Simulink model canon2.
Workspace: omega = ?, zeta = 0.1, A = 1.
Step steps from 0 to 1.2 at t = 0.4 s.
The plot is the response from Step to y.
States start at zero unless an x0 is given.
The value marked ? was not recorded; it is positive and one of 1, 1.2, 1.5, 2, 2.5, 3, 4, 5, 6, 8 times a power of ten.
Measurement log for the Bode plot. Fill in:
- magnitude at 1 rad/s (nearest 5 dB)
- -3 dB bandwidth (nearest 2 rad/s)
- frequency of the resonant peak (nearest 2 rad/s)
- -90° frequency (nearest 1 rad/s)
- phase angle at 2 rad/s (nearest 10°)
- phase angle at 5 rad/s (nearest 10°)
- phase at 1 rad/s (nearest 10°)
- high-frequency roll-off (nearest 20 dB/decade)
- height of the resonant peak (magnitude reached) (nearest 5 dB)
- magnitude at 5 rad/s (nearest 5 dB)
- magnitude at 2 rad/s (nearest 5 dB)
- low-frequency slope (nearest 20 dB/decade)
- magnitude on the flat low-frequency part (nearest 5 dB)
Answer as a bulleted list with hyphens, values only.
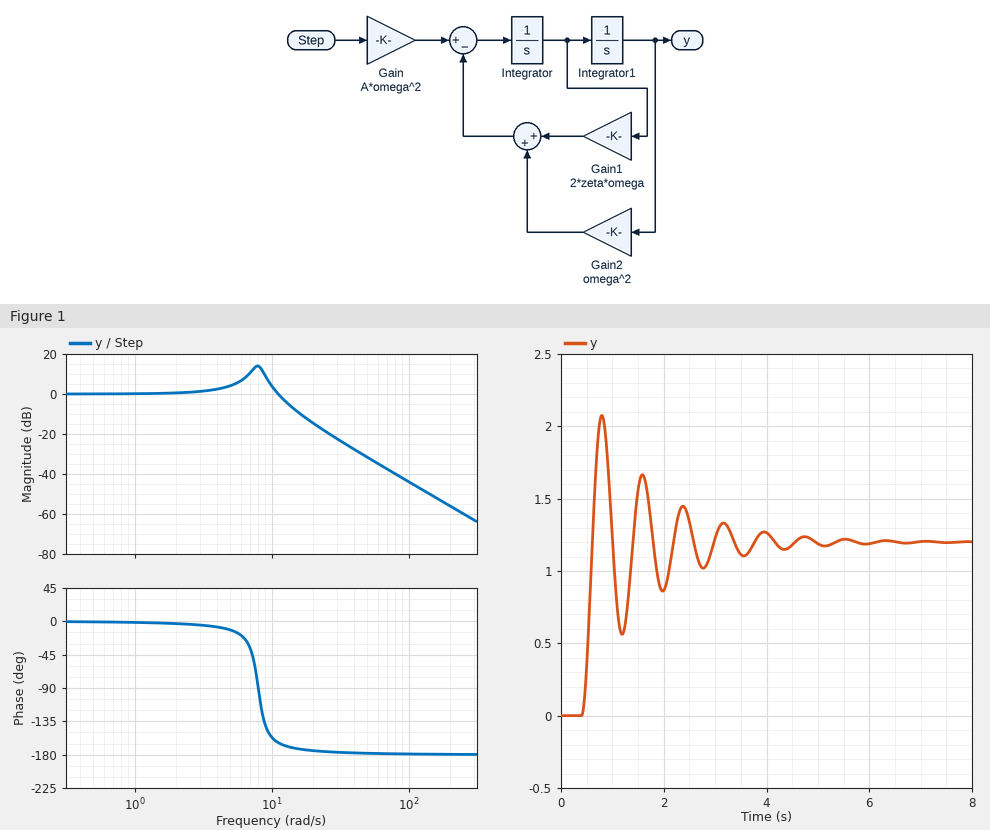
- 0 dB
- 12 rad/s
- 8 rad/s
- 8 rad/s
- 0°
- -10°
- 0°
- -40 dB/decade
- 15 dB
- 5 dB
- 0 dB
- 0 dB/decade
- 0 dB
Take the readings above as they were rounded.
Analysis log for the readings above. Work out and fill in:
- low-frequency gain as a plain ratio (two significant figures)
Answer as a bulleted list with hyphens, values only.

- 1.0
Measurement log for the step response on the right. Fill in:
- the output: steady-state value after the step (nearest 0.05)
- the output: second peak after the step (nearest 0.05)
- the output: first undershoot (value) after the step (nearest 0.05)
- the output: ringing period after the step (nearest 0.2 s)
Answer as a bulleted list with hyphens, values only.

- 1.20
- 1.65
- 0.55
- 0.8 s
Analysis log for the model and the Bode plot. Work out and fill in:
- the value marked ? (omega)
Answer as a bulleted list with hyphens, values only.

- 8
